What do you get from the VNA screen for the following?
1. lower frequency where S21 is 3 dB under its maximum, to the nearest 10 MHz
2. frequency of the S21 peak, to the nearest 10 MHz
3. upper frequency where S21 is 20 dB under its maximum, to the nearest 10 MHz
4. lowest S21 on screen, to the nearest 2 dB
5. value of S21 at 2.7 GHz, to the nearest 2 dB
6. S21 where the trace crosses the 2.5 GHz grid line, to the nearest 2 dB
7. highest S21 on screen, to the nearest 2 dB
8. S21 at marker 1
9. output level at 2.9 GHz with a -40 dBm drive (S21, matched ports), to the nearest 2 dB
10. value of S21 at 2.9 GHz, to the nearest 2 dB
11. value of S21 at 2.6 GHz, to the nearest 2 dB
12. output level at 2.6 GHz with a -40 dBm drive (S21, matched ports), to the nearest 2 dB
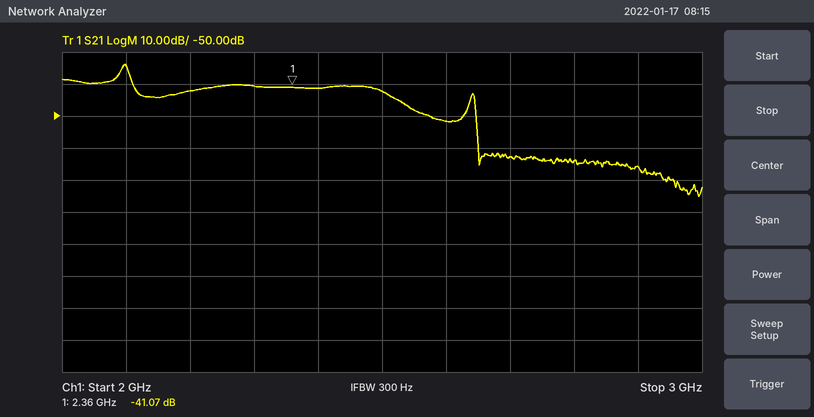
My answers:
2.09 GHz
2.10 GHz
2.65 GHz
-76 dB
-62 dB
-42 dB
-34 dB
-41.07 dB
-106 dBm
-66 dB
-52 dB
-92 dBm
